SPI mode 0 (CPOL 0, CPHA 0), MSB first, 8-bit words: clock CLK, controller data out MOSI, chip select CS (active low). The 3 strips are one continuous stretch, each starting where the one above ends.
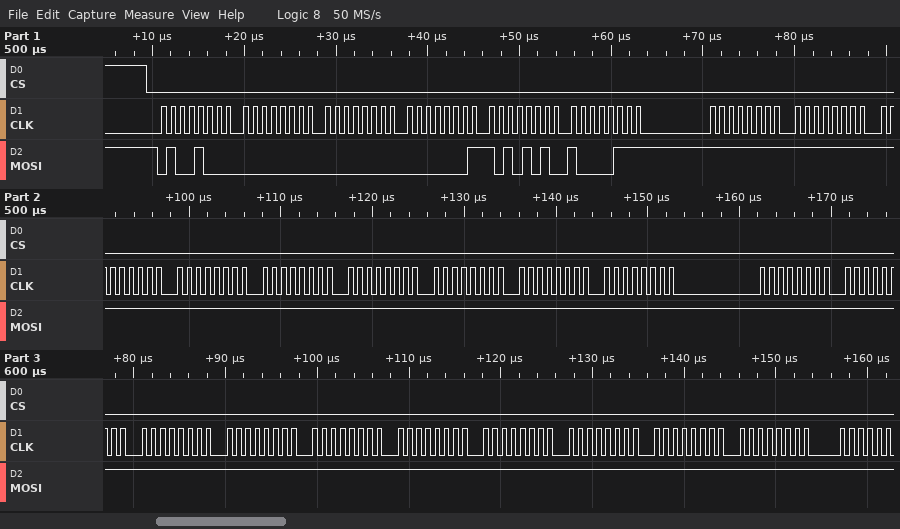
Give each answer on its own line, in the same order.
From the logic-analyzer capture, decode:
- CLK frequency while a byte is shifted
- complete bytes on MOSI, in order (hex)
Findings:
1 MHz
48 00 00 01 AA 87 FF FF FF FF FF FF FF FF FF FF FF FF FF FF FF FF FF FF FF
